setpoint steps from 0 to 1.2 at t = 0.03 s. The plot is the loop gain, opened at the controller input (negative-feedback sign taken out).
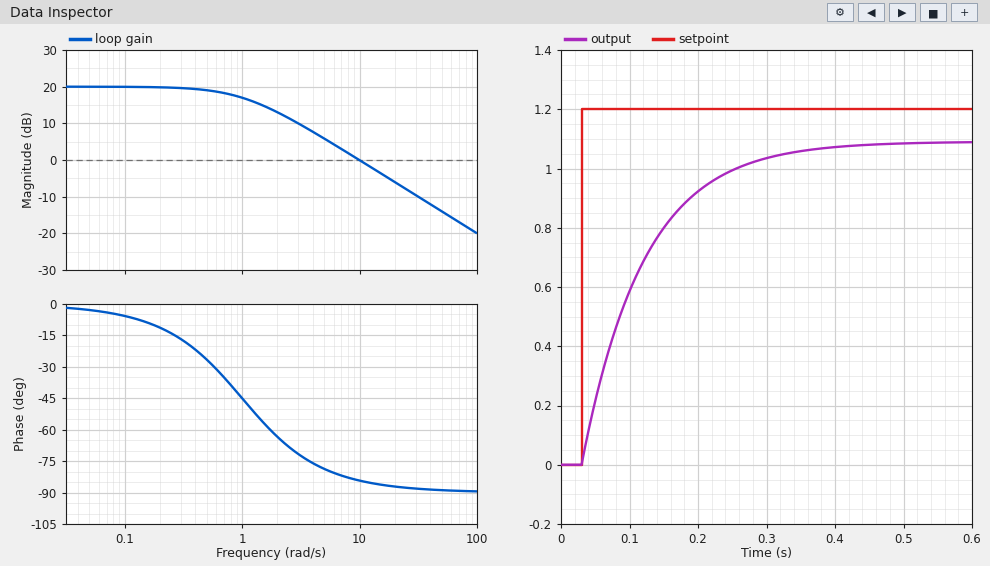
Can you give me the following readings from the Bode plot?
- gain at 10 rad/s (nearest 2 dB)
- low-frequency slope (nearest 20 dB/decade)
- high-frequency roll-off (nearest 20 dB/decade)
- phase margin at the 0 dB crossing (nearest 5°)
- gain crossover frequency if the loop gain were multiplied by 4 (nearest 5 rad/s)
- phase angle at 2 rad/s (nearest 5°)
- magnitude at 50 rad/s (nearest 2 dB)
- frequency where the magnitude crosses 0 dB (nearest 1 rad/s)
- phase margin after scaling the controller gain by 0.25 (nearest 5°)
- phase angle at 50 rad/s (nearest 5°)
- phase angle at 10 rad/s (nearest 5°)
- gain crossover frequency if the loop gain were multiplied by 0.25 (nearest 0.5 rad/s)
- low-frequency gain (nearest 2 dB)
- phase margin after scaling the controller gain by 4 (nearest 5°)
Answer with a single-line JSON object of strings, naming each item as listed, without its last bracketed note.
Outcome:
{"gain at 10 rad/s": "0 dB", "low-frequency slope": "0 dB/decade", "high-frequency roll-off": "-20 dB/decade", "phase margin at the 0 dB crossing": "95°", "gain crossover frequency if the loop gain were multiplied by 4": "40 rad/s", "phase angle at 2 rad/s": "-65°", "magnitude at 50 rad/s": "-14 dB", "frequency where the magnitude crosses 0 dB": "10 rad/s", "phase margin after scaling the controller gain by 0.25": "115°", "phase angle at 50 rad/s": "-90°", "phase angle at 10 rad/s": "-85°", "gain crossover frequency if the loop gain were multiplied by 0.25": "2.5 rad/s", "low-frequency gain": "20 dB", "phase margin after scaling the controller gain by 4": "90°"}
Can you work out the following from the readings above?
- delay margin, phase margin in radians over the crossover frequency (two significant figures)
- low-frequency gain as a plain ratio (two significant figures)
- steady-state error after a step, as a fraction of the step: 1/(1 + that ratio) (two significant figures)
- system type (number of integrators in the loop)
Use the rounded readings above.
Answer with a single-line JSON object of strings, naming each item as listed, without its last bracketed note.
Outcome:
{"delay margin, phase margin in radians over the crossover frequency": "0.17 s", "low-frequency gain as a plain ratio": "10", "steady-state error after a step, as a fraction of the step: 1/(1 + that ratio)": "0.091", "system type": "0"}
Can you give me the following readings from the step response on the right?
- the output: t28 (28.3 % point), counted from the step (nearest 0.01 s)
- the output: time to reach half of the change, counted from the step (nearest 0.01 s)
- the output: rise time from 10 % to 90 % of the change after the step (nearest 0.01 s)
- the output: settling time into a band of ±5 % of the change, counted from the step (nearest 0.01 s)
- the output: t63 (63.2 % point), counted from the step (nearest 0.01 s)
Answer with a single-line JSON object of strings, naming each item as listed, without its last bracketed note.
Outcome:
{"the output: t28 (28.3 % point), counted from the step": "0.03 s", "the output: time to reach half of the change, counted from the step": "0.06 s", "the output: rise time from 10 % to 90 % of the change after the step": "0.20 s", "the output: settling time into a band of ±5 % of the change, counted from the step": "0.27 s", "the output: t63 (63.2 % point), counted from the step": "0.09 s"}
